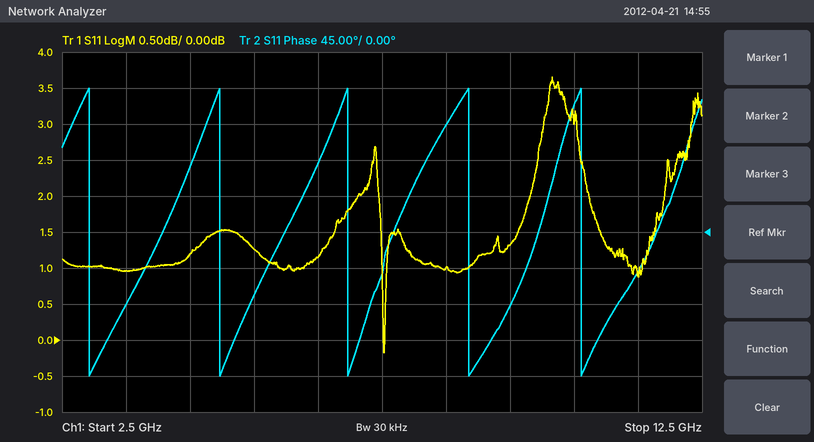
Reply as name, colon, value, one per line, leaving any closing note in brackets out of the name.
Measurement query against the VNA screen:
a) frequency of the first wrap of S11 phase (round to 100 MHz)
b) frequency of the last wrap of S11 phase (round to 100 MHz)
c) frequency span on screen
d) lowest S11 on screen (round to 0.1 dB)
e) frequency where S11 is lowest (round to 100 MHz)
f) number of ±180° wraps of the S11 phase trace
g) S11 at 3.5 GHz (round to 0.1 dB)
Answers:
frequency of the first wrap of S11 phase: 2.9 GHz
frequency of the last wrap of S11 phase: 10.6 GHz
frequency span on screen: 10 GHz
lowest S11 on screen: -0.2 dB
frequency where S11 is lowest: 7.5 GHz
number of ±180° wraps of the S11 phase trace: 5
S11 at 3.5 GHz: 1.0 dB
